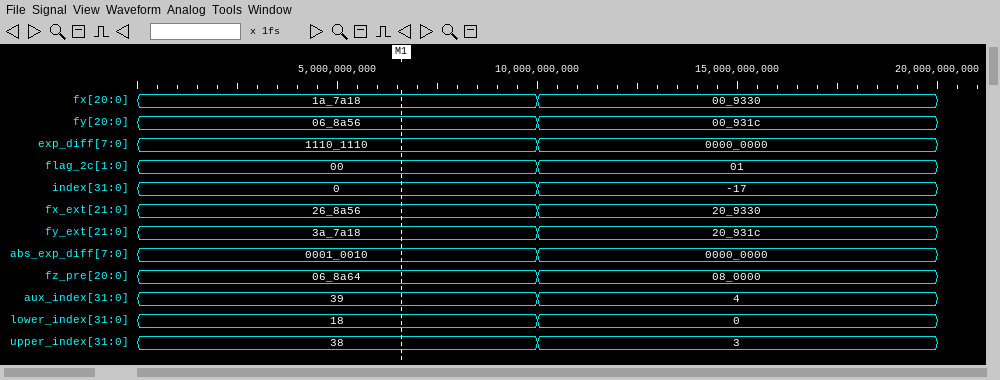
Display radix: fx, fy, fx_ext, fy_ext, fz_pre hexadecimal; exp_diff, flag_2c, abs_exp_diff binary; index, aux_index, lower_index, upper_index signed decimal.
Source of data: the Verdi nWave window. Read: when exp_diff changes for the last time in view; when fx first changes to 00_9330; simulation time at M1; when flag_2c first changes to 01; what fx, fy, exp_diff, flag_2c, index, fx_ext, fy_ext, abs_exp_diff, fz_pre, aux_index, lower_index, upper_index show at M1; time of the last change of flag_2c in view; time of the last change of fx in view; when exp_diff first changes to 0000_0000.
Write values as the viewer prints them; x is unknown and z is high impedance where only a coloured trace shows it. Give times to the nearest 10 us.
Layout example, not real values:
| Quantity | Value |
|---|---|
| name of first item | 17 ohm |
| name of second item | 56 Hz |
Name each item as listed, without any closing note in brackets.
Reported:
| Quantity | Value |
|---|---|
| when exp_diff changes for the last time in view | 10 us |
| when fx first changes to 00_9330 | 10 us |
| simulation time at M1 | 10 us |
| when flag_2c first changes to 01 | 10 us |
| what fx, fy, exp_diff, flag_2c, index, fx_ext, fy_ext, abs_exp_diff, fz_pre, aux_index, lower_index, upper_index show at M1 | fx=1a_7a18, fy=06_8a56, exp_diff=1110_1110, flag_2c=00, index=0, fx_ext=26_8a56, fy_ext=3a_7a18, abs_exp_diff=0001_0010, fz_pre=06_8a64, aux_index=39, lower_index=18, upper_index=38 |
| time of the last change of flag_2c in view | 10 us |
| time of the last change of fx in view | 10 us |
| when exp_diff first changes to 0000_0000 | 10 us |
